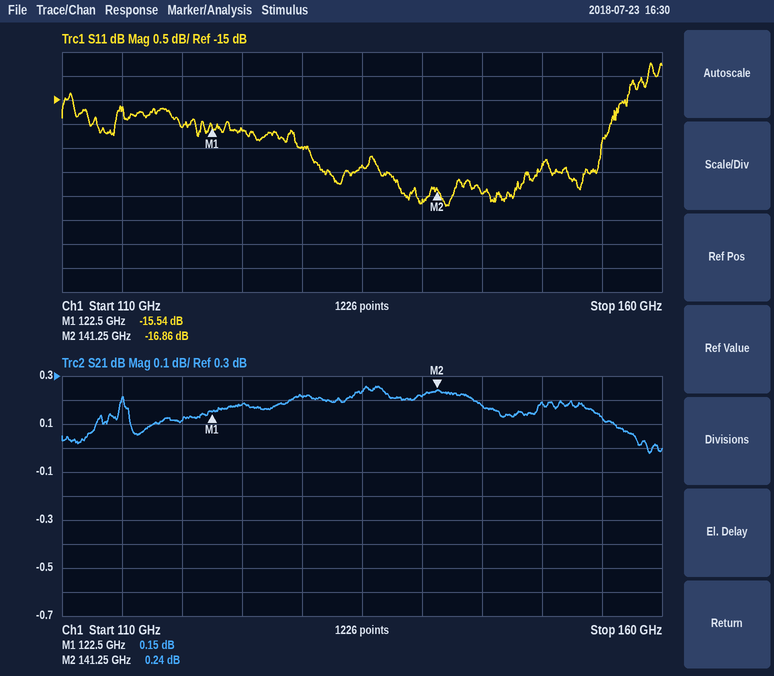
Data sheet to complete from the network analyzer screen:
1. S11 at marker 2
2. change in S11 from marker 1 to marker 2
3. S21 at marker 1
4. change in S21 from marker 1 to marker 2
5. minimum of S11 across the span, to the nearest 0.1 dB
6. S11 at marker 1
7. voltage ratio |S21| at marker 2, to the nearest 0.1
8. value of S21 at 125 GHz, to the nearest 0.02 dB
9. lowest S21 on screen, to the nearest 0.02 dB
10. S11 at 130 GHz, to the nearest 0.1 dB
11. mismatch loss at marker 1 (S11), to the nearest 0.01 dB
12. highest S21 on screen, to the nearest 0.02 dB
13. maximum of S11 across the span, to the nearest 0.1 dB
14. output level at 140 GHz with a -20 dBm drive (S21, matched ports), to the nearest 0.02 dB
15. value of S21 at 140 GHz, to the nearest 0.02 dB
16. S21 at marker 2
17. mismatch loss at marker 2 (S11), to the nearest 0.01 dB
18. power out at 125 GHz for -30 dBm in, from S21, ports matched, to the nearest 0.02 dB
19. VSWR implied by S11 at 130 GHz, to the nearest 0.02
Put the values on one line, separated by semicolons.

-16.86 dB; -1.32 dB; 0.15 dB; 0.09 dB; -17.2 dB; -15.54 dB; 1.0; 0.18 dB; -0.02 dB; -16.0 dB; 0.12 dB; 0.26 dB; -14.2 dB; -19.78 dBm; 0.22 dB; 0.24 dB; 0.09 dB; -29.82 dBm; 1.38
